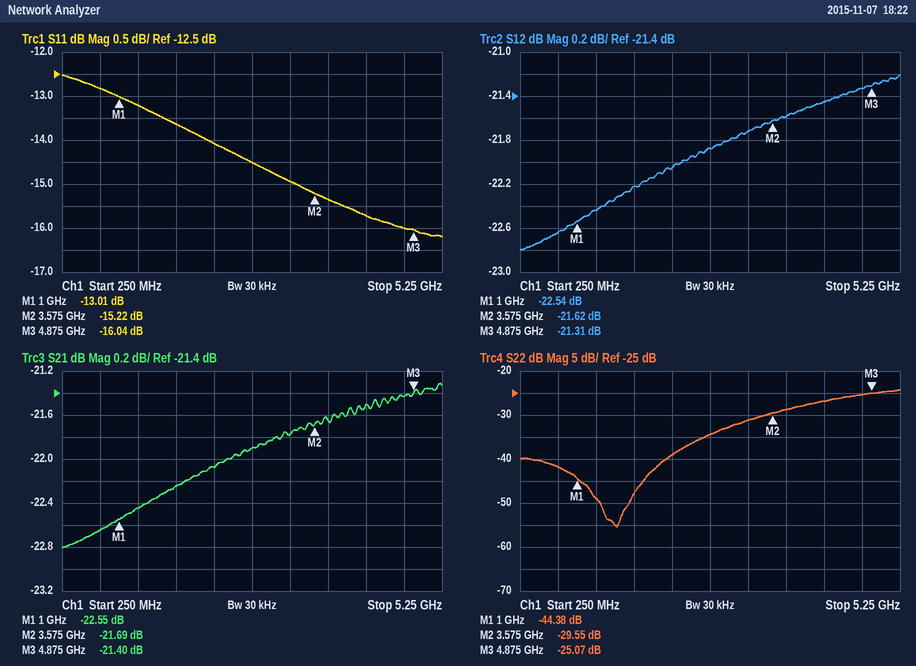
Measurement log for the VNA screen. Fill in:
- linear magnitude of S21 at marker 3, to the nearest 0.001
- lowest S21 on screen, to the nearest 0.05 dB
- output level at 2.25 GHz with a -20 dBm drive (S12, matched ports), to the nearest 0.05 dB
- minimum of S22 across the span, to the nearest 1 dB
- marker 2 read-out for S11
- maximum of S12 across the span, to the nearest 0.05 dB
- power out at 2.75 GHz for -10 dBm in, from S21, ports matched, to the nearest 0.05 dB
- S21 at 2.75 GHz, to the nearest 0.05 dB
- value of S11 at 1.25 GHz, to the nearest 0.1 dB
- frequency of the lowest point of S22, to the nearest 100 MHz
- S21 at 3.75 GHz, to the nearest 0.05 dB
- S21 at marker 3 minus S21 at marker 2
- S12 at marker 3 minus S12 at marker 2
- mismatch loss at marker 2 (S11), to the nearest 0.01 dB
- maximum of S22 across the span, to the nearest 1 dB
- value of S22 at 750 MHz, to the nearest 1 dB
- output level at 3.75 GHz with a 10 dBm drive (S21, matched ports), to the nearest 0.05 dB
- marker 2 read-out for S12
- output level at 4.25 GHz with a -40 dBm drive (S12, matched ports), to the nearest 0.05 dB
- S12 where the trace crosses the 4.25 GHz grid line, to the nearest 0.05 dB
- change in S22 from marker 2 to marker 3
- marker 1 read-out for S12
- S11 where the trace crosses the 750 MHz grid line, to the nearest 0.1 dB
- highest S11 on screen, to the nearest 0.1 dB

0.085
-22.80 dB
-42.05 dBm
-55 dB
-15.22 dB
-21.20 dB
-31.90 dBm
-21.90 dB
-13.2 dB
1.5 GHz
-21.65 dB
0.29 dB
0.31 dB
0.13 dB
-24 dB
-42 dB
-11.65 dBm
-21.62 dB
-61.45 dBm
-21.45 dB
4.48 dB
-22.54 dB
-12.8 dB
-12.5 dB
